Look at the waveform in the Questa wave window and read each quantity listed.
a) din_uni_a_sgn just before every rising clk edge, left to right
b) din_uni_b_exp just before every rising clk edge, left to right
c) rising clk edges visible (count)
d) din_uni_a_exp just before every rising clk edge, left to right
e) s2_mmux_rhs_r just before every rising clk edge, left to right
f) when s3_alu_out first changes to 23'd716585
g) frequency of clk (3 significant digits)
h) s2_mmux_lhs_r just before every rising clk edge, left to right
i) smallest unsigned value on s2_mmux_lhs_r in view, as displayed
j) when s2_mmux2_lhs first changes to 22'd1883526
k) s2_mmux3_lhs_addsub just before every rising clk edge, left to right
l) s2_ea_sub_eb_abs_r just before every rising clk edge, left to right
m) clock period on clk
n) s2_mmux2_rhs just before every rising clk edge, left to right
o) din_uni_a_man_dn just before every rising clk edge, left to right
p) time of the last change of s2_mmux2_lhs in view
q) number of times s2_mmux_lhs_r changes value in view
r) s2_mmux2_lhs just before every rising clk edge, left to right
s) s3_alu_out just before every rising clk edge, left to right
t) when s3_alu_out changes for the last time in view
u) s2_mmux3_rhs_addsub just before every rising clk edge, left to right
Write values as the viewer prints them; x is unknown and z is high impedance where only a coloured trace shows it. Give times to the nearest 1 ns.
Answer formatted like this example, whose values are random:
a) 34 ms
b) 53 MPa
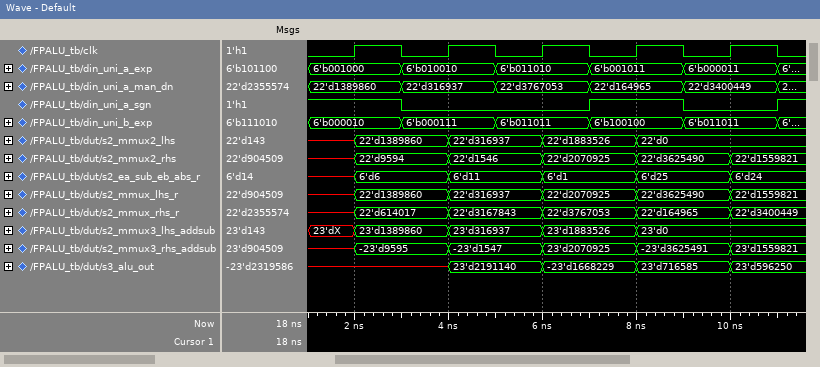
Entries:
a) 1 0 0 1 0
b) 6'b000010, 6'b000111, 6'b011011, 6'b100100, 6'b011011
c) 5
d) 6'b001000, 6'b010010, 6'b011010, 6'b001011, 6'b000011
e) x, 22'd614017, 22'd3167843, 22'd3767053, 22'd164965
f) 8 ns
g) 500 MHz
h) x, 22'd1389860, 22'd316937, 22'd2070925, 22'd3625490
i) 22'd316937
j) 6 ns
k) 23'dX, 23'd1389860, 23'd316937, 23'd1883526, 23'd0
l) x, 6'd6, 6'd11, 6'd1, 6'd25
m) 2 ns
n) x, 22'd9594, 22'd1546, 22'd2070925, 22'd3625490
o) 22'd1389860, 22'd316937, 22'd3767053, 22'd164965, 22'd3400449
p) 8 ns
q) 5
r) x, 22'd1389860, 22'd316937, 22'd1883526, 22'd0
s) x, x, 23'd2191140, -23'd1668229, 23'd716585
t) 10 ns
u) x, -23'd9595, -23'd1547, 23'd2070925, -23'd3625491
